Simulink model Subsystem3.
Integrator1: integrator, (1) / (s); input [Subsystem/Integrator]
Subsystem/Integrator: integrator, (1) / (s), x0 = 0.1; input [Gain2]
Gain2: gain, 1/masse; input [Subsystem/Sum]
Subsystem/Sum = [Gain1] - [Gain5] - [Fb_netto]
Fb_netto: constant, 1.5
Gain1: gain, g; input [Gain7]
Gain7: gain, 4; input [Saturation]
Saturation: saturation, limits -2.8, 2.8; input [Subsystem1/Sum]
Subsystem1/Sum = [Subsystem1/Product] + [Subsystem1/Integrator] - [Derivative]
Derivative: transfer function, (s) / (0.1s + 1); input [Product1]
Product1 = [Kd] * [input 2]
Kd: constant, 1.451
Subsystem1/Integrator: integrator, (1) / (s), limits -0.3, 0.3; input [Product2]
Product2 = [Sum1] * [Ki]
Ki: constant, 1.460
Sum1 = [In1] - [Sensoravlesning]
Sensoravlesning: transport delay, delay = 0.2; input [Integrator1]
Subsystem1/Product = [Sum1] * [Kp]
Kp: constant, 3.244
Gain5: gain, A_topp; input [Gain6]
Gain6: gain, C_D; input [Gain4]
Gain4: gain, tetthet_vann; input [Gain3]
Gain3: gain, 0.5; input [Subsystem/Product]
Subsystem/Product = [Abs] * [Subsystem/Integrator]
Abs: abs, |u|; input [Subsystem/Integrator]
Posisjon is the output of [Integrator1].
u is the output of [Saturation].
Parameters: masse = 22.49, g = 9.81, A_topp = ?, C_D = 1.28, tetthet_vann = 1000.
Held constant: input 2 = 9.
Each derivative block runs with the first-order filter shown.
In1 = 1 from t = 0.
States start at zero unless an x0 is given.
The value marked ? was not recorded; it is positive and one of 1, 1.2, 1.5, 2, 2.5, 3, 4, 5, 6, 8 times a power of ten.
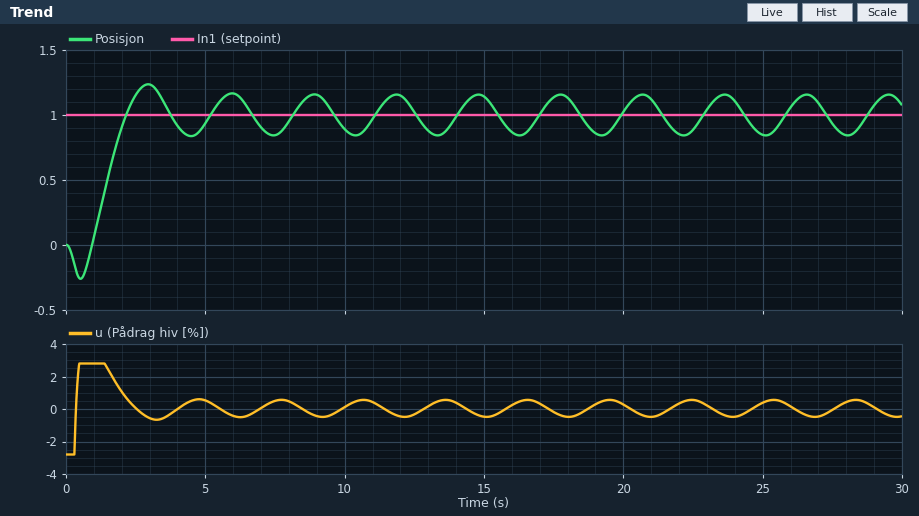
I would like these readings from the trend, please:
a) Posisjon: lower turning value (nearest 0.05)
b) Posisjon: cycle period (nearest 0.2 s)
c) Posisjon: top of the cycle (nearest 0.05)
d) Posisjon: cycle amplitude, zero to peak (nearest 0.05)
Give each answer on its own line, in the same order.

0.85
3.0 s
1.15
0.15
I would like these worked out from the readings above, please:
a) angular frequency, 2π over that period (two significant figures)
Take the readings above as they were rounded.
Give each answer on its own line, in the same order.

2.1 rad/s
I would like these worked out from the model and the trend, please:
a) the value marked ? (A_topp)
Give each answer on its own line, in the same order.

0.2
